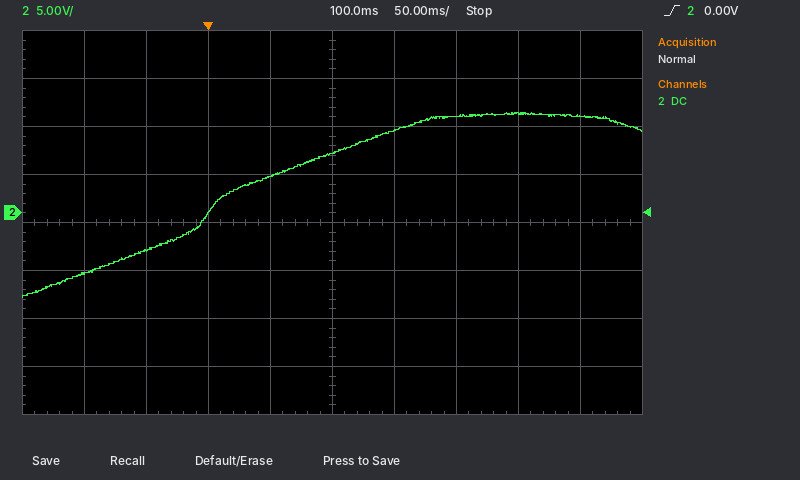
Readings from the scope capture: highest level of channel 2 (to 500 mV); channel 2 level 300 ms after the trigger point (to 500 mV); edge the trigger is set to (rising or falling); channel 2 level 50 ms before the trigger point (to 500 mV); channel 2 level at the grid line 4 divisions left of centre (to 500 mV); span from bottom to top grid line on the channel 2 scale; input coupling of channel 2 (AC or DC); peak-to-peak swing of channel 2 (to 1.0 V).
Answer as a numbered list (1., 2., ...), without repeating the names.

1. 10.5 V
2. 10.0 V
3. rising
4. -4.0 V
5. -6.5 V
6. 40 V
7. DC
8. 19.0 V
